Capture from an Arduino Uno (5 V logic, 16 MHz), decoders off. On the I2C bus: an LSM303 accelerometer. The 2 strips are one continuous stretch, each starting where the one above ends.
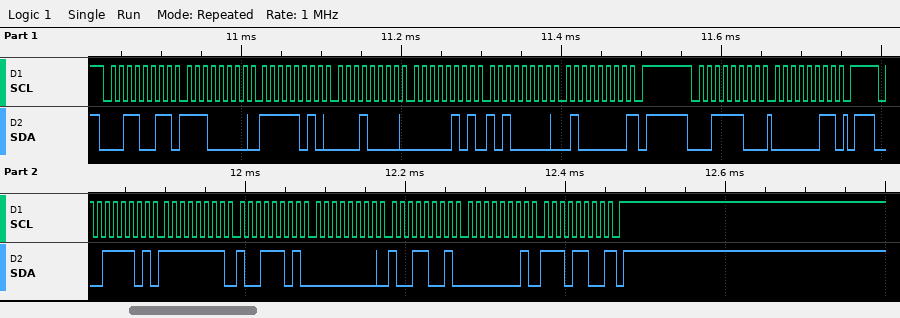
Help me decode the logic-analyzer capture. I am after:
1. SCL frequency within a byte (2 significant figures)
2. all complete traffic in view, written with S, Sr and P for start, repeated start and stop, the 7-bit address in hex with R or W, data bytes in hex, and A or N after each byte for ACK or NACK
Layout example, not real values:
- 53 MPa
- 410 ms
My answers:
- 100 kHz
- S 19R A E0 A FA A 10 A 05 A A0 A 40 N P S 1EW A 03 A P S 1ER A FF A 9D A 00 A 99 A 01 A EC N P
